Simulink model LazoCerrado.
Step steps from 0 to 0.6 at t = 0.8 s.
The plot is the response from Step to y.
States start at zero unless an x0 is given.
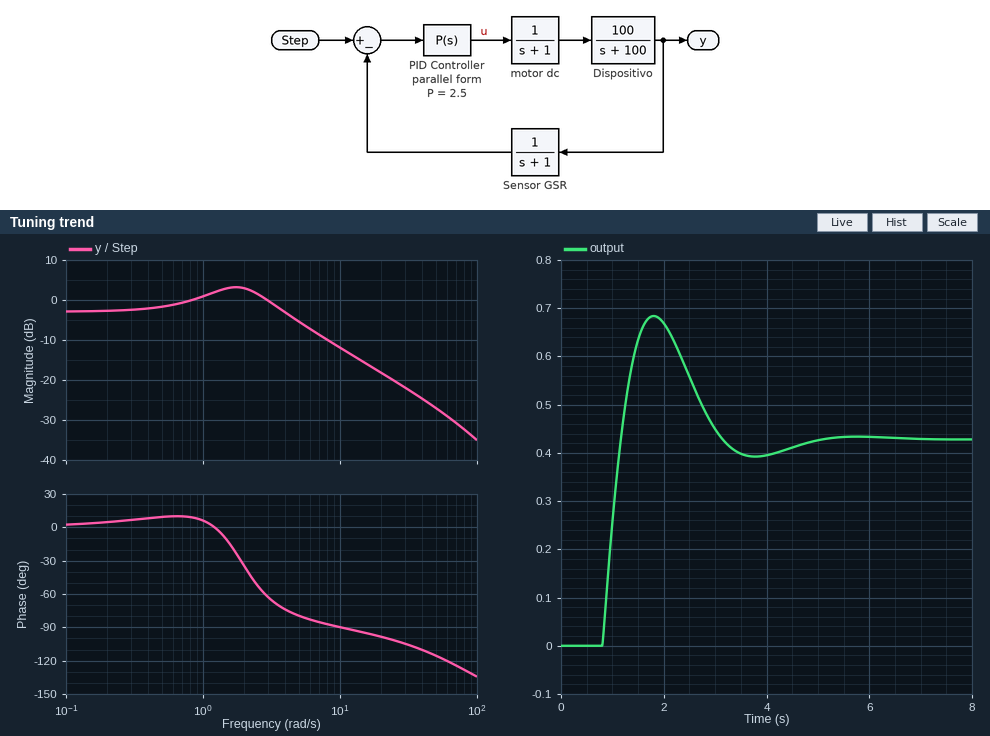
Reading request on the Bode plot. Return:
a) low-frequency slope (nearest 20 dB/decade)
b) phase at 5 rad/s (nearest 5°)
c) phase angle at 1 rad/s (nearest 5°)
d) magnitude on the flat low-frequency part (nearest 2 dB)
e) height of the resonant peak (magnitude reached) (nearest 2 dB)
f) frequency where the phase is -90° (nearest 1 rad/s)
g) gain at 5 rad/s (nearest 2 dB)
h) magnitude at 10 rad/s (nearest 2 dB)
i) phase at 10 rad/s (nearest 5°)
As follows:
0 dB/decade
-80°
5°
-2 dB
4 dB
10 rad/s
-6 dB
-12 dB
-90°
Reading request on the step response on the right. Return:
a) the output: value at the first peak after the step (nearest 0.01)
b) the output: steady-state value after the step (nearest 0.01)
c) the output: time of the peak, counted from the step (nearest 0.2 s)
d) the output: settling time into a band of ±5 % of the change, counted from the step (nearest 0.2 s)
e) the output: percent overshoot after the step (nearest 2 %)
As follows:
0.68
0.43
1.0 s
3.6 s
60 %
